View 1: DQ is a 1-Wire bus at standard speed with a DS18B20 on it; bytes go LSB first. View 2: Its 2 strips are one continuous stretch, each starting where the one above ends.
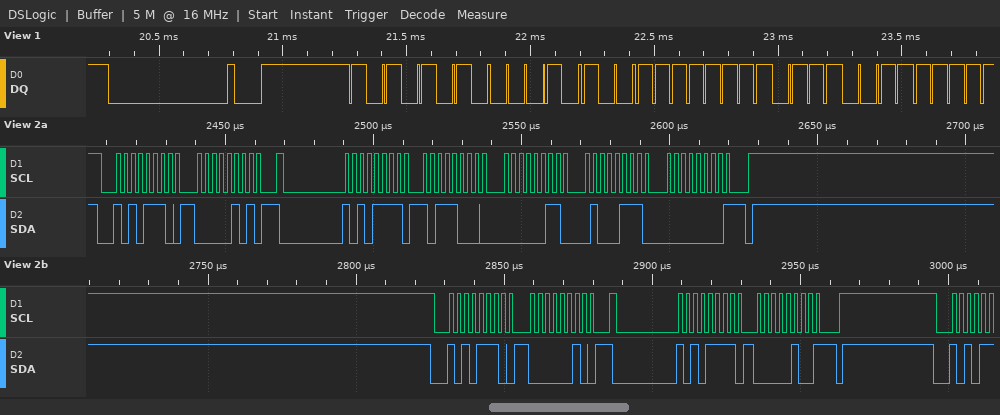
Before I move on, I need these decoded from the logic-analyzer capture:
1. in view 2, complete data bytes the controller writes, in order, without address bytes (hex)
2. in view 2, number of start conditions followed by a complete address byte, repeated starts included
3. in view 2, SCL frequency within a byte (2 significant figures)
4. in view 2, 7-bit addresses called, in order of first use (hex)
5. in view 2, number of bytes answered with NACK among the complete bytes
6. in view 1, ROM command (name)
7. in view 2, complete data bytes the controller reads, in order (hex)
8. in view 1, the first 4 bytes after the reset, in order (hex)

05 02
4
400 kHz
0x57
2
Match ROM
B8 03 47 00 04
55 28 FF CE
